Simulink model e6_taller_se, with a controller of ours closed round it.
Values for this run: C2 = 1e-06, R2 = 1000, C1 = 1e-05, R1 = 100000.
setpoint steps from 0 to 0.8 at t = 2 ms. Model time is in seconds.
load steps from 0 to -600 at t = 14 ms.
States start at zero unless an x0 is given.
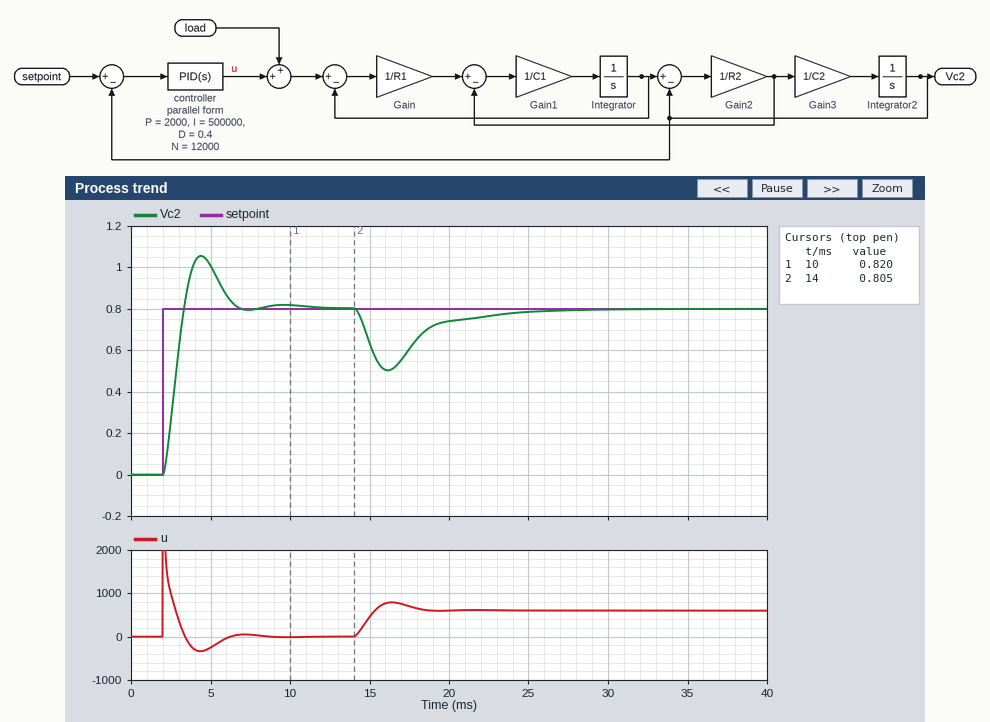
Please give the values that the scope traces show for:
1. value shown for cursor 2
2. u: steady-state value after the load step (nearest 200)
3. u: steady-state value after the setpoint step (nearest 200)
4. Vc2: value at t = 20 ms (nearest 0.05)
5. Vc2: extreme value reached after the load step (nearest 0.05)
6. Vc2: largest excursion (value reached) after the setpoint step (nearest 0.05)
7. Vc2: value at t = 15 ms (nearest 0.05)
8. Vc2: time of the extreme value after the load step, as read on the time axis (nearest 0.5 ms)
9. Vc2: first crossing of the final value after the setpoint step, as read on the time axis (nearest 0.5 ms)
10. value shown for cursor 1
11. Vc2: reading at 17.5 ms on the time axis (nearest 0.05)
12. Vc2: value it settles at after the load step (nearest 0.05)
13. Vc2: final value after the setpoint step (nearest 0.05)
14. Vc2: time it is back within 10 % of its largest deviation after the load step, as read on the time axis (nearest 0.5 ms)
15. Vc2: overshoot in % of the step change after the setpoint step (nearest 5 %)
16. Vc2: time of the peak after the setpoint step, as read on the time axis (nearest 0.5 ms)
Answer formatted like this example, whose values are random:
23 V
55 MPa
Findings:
0.805
600
0
0.75
0.50
1.05
0.65
16.0 ms
3.5 ms
0.820
0.60
0.80
0.80
23.0 ms
30 %
4.5 ms
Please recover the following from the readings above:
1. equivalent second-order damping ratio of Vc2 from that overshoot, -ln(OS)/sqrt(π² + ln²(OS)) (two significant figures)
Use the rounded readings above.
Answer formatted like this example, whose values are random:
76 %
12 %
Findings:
0.36
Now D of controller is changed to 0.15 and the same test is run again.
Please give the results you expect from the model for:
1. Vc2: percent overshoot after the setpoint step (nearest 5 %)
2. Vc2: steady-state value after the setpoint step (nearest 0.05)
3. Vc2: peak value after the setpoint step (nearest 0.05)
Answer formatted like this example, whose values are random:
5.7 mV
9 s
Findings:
40 %
0.80
1.15
